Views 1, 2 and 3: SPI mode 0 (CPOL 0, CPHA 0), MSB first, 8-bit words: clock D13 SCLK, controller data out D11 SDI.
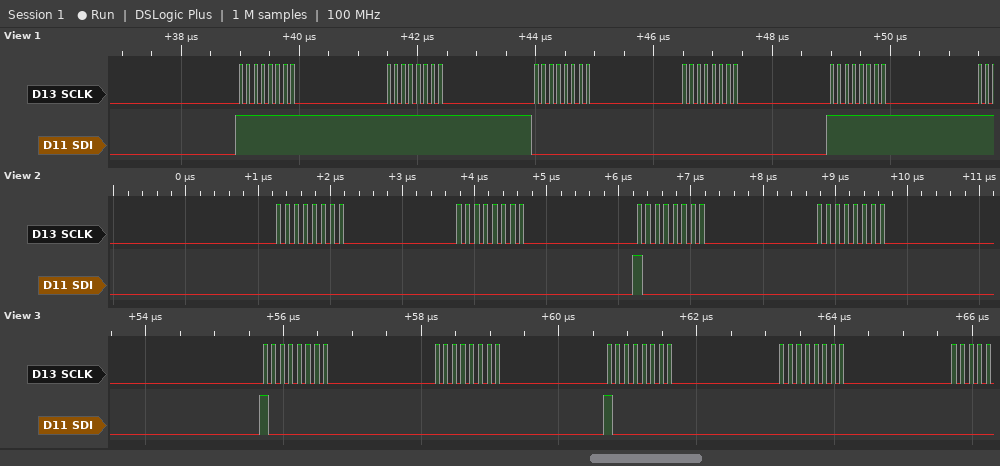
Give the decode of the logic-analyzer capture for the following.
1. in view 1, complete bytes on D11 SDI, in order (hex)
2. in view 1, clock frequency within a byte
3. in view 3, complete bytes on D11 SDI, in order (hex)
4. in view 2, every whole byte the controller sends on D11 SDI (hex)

FF FF 00 00 FF
8 MHz
0x80 0x00 0x80 0x00
00 00 80 00
